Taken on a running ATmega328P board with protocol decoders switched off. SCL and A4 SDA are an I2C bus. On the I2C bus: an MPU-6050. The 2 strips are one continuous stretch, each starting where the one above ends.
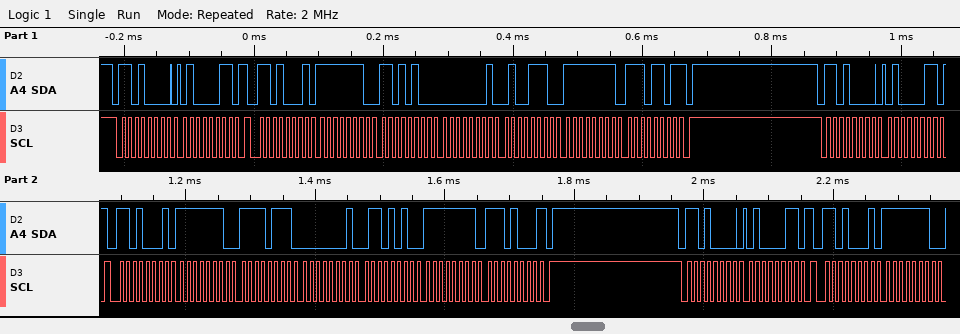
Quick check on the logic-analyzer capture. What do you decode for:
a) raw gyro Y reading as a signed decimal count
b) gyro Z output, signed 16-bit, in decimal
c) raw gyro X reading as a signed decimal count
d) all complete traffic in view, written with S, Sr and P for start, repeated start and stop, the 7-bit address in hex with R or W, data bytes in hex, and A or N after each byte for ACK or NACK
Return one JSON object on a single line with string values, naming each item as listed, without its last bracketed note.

{"raw gyro Y reading as a signed decimal count": "334", "gyro Z output, signed 16-bit, in decimal": "-19", "raw gyro X reading as a signed decimal count": "-300", "all complete traffic in view, written with S, Sr and P for start, repeated start and stop, the 7-bit address in hex with R or W, data bytes in hex, and A or N after each byte for ACK or NACK": "S 68W A 43 A Sr 68R A FE A D4 A 01 A 4E A FF A ED N P S 68W A 43 A Sr 68R A FE A F7 A 01 A 6A A FF A E8 N P S 68W A 43 A Sr 68R A FE A"}
